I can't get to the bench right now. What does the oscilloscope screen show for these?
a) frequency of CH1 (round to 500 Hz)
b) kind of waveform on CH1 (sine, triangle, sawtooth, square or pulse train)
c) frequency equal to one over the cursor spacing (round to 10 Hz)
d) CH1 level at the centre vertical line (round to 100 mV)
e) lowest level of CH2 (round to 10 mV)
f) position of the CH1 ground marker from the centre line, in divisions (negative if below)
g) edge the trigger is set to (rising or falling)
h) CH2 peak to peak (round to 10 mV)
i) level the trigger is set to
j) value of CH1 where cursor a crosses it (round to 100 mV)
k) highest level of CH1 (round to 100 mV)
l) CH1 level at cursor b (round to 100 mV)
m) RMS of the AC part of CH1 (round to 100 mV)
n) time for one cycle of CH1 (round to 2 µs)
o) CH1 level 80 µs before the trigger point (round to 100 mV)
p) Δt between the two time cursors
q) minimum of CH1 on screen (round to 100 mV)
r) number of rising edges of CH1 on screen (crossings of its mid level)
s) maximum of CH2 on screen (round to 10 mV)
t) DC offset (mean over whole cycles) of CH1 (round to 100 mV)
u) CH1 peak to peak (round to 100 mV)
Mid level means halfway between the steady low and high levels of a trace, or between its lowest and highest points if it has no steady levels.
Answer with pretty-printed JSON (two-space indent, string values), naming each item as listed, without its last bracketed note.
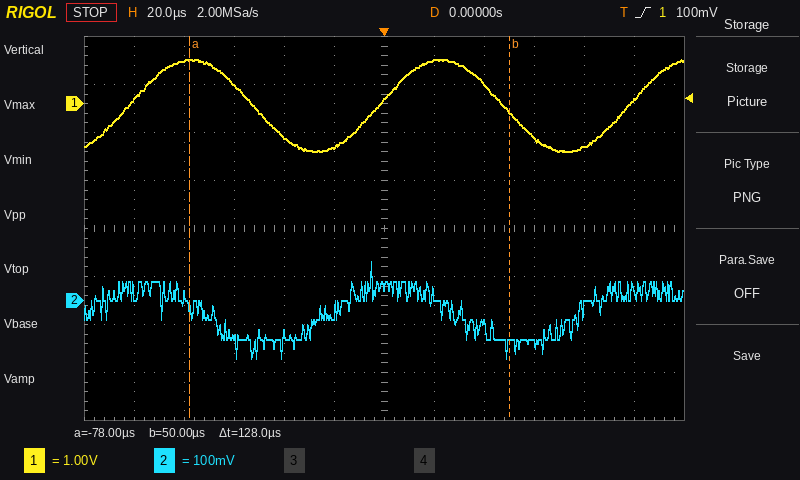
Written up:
{
  "frequency of CH1": "10.0 kHz",
  "kind of waveform on CH1": "sine",
  "frequency equal to one over the cursor spacing": "7.81 kHz",
  "CH1 level at the centre vertical line": "100 mV",
  "lowest level of CH2": "-120 mV",
  "position of the CH1 ground marker from the centre line, in divisions": "+2.6 div",
  "edge the trigger is set to": "rising",
  "CH2 peak to peak": "200 mV",
  "level the trigger is set to": "100 mV",
  "value of CH1 where cursor a crosses it": "900 mV",
  "highest level of CH1": "900 mV",
  "CH1 level at cursor b": "-200 mV",
  "RMS of the AC part of CH1": "700 mV",
  "time for one cycle of CH1": "100 µs",
  "CH1 level 80 µs before the trigger point": "900 mV",
  "Δt between the two time cursors": "128 µs",
  "minimum of CH1 on screen": "-1.0 V",
  "number of rising edges of CH1 on screen": "3",
  "maximum of CH2 on screen": "80 mV",
  "DC offset (mean over whole cycles) of CH1": "0.0 V",
  "CH1 peak to peak": "1.9 V"
}
